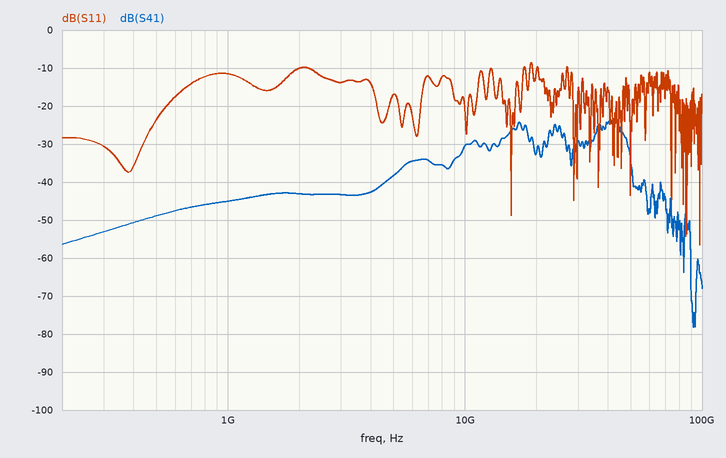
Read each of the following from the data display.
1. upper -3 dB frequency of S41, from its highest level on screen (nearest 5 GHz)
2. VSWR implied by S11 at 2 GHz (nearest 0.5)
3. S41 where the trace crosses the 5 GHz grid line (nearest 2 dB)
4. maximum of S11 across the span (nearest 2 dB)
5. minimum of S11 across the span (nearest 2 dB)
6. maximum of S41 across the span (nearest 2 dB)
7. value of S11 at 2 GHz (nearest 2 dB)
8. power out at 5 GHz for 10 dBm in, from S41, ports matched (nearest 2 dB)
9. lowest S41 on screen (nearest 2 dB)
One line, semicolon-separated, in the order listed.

45 GHz; 2.0; -38 dB; -8 dB; -56 dB; -24 dB; -10 dB; -28 dBm; -78 dB
